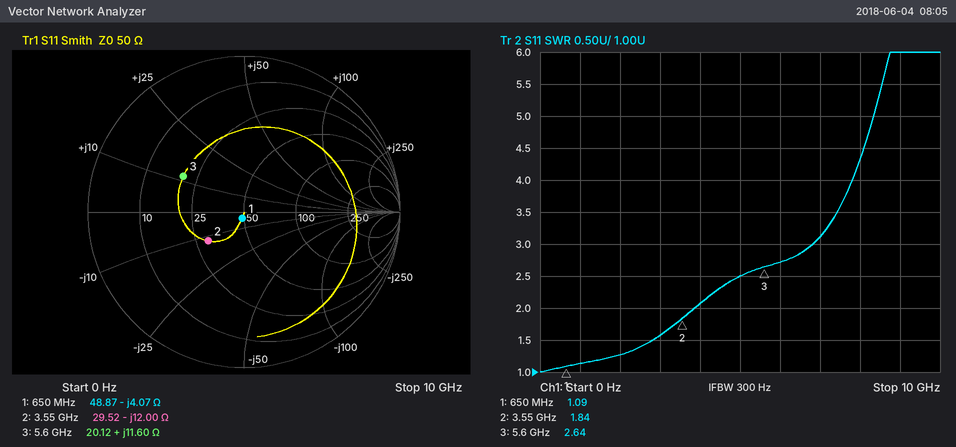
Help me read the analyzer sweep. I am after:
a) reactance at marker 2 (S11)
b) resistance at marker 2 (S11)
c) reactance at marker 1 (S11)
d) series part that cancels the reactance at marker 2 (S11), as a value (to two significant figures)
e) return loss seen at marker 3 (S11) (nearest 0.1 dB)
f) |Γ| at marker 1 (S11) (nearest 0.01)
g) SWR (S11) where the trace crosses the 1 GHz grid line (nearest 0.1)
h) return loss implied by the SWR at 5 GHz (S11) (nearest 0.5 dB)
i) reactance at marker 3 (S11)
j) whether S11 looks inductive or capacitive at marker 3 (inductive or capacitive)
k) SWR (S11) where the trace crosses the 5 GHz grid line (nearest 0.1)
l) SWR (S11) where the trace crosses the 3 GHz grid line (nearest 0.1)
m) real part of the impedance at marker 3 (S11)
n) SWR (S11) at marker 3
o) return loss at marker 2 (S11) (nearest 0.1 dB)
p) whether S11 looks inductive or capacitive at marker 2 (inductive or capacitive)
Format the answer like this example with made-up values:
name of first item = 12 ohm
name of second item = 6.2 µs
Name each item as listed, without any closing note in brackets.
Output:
reactance at marker 2 = -12.00 Ω
resistance at marker 2 = 29.52 Ω
reactance at marker 1 = -4.07 Ω
series part that cancels the reactance at marker 2 (S11), as a value = 540 pH
return loss seen at marker 3 (S11) = 6.9 dB
|Γ| at marker 1 (S11) = 0.04
SWR (S11) where the trace crosses the 1 GHz grid line = 1.1
return loss implied by the SWR at 5 GHz (S11) = 7.5 dB
reactance at marker 3 = +11.60 Ω
whether S11 looks inductive or capacitive at marker 3 = inductive
SWR (S11) where the trace crosses the 5 GHz grid line = 2.5
SWR (S11) where the trace crosses the 3 GHz grid line = 1.6
real part of the impedance at marker 3 = 20.12 Ω
SWR (S11) at marker 3 = 2.64
return loss at marker 2 (S11) = 10.6 dB
whether S11 looks inductive or capacitive at marker 2 = capacitive
